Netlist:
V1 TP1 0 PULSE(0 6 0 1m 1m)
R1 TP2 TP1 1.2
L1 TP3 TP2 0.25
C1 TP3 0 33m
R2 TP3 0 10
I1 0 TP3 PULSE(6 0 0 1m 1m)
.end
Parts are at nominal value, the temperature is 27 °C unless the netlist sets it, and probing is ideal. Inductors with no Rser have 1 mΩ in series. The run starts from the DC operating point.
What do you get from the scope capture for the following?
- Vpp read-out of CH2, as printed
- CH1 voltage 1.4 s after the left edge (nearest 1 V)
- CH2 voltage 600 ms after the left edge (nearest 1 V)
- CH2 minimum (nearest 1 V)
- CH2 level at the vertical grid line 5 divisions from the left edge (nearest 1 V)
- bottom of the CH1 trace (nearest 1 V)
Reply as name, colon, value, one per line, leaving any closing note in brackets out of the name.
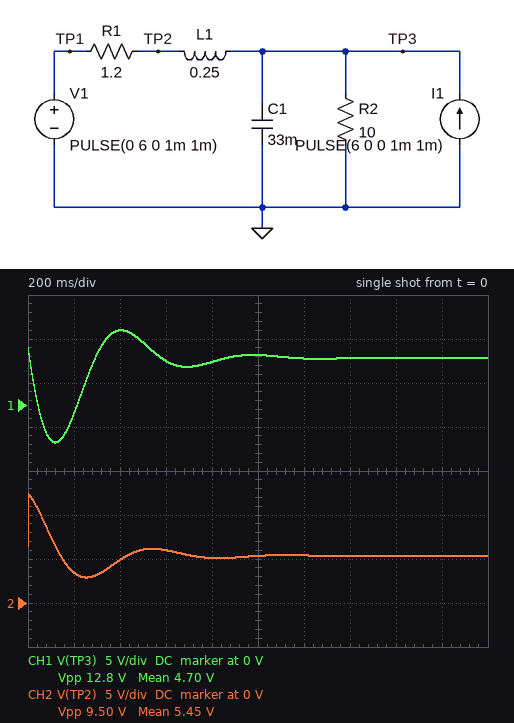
Vpp read-out of CH2, as printed: 9.50 V
CH1 voltage 1.4 s after the left edge: 5 V
CH2 voltage 600 ms after the left edge: 6 V
CH2 minimum: 3 V
CH2 level at the vertical grid line 5 divisions from the left edge: 5 V
bottom of the CH1 trace: -4 V
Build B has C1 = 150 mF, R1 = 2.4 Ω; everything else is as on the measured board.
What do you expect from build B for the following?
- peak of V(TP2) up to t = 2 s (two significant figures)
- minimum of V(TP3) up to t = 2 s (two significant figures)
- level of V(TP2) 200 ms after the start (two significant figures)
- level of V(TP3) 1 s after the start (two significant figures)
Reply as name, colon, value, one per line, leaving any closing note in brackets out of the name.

peak of V(TP2) up to t = 2 s: 18 V
minimum of V(TP3) up to t = 2 s: 4.7 V
level of V(TP2) 200 ms after the start: 9.4 V
level of V(TP3) 1 s after the start: 4.8 V
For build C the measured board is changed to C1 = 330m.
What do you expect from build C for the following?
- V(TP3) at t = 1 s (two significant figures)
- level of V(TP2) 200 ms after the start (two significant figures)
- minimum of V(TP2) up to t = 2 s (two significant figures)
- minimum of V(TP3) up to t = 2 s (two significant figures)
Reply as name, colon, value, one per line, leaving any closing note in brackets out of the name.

V(TP3) at t = 1 s: 5.1 V
level of V(TP2) 200 ms after the start: 7.8 V
minimum of V(TP2) up to t = 2 s: 4.4 V
minimum of V(TP3) up to t = 2 s: 3.7 V
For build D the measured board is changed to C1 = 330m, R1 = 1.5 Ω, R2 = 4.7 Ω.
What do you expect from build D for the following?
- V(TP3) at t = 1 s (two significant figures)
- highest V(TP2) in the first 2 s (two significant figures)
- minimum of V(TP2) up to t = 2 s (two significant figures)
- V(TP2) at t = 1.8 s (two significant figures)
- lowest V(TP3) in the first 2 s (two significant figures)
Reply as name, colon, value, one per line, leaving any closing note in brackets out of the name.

V(TP3) at t = 1 s: 4.4 V
highest V(TP2) in the first 2 s: 13 V
minimum of V(TP2) up to t = 2 s: 4.2 V
V(TP2) at t = 1.8 s: 4.5 V
lowest V(TP3) in the first 2 s: 3.9 V
